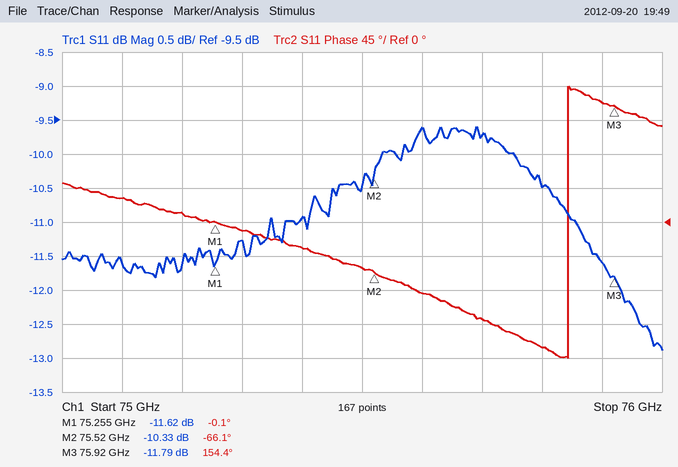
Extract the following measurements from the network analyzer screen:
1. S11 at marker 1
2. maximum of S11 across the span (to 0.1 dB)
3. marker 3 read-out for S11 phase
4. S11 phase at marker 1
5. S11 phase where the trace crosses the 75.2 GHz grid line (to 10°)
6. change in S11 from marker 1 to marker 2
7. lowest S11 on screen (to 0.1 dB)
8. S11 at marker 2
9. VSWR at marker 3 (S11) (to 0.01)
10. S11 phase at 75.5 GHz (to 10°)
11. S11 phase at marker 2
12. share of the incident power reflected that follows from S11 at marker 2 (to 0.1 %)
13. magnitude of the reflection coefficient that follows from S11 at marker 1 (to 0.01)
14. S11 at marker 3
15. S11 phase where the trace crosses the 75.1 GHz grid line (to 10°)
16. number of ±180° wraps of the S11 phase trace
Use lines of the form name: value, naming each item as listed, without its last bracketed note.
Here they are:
S11 at marker 1: -11.62 dB
maximum of S11 across the span: -9.6 dB
marker 3 read-out for S11 phase: 154.4°
S11 phase at marker 1: -0.1°
S11 phase where the trace crosses the 75.2 GHz grid line: 10°
change in S11 from marker 1 to marker 2: 1.29 dB
lowest S11 on screen: -12.9 dB
S11 at marker 2: -10.33 dB
VSWR at marker 3 (S11): 1.69
S11 phase at 75.5 GHz: -60°
S11 phase at marker 2: -66.1°
share of the incident power reflected that follows from S11 at marker 2: 9.3 %
magnitude of the reflection coefficient that follows from S11 at marker 1: 0.26
S11 at marker 3: -11.79 dB
S11 phase where the trace crosses the 75.1 GHz grid line: 30°
number of ±180° wraps of the S11 phase trace: 1
